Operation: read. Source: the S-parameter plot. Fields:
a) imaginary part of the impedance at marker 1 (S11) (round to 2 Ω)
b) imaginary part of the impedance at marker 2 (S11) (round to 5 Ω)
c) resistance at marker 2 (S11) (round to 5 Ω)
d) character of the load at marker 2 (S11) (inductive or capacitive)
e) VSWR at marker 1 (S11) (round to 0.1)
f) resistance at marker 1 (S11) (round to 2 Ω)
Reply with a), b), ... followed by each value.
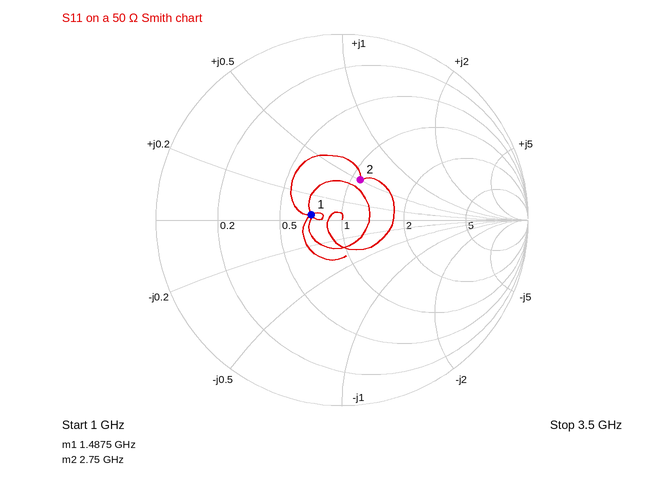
a) +2 Ω
b) +25 Ω
c) 55 Ω
d) inductive
e) 1.4
f) 36 Ω
